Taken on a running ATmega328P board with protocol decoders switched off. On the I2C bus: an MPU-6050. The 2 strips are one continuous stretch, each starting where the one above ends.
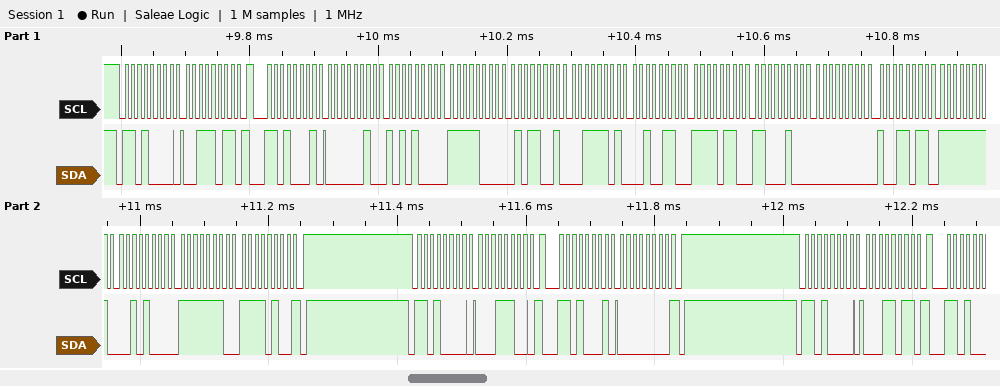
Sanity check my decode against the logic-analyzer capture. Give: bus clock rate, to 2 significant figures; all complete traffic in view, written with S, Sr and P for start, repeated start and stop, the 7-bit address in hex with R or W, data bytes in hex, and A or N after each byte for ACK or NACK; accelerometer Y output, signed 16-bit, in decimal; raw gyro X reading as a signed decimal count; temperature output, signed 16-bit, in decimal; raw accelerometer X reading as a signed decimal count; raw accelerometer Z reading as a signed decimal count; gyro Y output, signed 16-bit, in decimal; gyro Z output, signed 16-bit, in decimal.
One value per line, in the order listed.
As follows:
100 kHz
S 68W A 3B A Sr 68R A 02 A A8 A F8 A 59 A 3D A 26 A F6 A C4 A 00 A 9B A FF A 28 A FE A F4 N P S 68W A 1C A Sr 68R A 00 N P S 68W A 1B A
-1959
155
-2364
680
15654
-216
-268
